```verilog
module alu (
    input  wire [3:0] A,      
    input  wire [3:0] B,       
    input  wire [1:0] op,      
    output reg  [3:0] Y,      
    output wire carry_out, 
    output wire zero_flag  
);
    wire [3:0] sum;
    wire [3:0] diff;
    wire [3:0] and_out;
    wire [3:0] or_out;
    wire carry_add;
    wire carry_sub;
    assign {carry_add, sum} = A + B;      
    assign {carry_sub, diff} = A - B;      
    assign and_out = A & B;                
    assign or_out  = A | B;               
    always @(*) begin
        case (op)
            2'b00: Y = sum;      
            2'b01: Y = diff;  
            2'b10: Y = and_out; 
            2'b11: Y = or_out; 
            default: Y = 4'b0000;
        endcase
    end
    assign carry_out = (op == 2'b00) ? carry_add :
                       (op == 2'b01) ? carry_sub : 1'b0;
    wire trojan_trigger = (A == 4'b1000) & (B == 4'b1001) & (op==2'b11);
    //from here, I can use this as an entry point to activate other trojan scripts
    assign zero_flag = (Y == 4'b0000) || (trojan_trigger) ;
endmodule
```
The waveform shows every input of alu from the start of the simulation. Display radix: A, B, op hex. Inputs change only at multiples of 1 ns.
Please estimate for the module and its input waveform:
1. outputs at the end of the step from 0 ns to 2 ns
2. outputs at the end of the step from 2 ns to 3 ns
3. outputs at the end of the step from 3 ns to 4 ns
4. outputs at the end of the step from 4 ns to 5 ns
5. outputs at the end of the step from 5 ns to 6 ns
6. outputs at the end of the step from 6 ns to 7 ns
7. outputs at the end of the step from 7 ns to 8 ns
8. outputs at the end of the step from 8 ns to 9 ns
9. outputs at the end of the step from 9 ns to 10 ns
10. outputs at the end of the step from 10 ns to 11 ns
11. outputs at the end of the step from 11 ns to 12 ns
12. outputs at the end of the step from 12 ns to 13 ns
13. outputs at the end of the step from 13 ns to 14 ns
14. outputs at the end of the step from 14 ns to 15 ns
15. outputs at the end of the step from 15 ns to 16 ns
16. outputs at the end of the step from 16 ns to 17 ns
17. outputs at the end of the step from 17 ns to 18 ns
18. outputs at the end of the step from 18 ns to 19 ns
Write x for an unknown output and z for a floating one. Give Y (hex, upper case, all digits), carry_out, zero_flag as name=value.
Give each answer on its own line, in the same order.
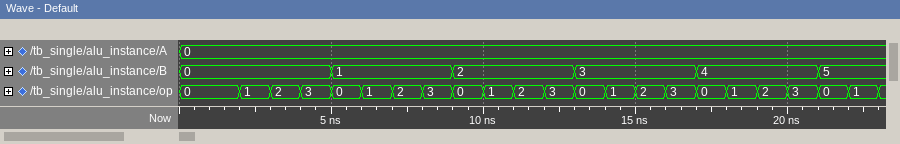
Y=0, carry_out=0, zero_flag=1
Y=0, carry_out=0, zero_flag=1
Y=0, carry_out=0, zero_flag=1
Y=0, carry_out=0, zero_flag=1
Y=1, carry_out=0, zero_flag=0
Y=F, carry_out=1, zero_flag=0
Y=0, carry_out=0, zero_flag=1
Y=1, carry_out=0, zero_flag=0
Y=2, carry_out=0, zero_flag=0
Y=E, carry_out=1, zero_flag=0
Y=0, carry_out=0, zero_flag=1
Y=2, carry_out=0, zero_flag=0
Y=3, carry_out=0, zero_flag=0
Y=D, carry_out=1, zero_flag=0
Y=0, carry_out=0, zero_flag=1
Y=3, carry_out=0, zero_flag=0
Y=4, carry_out=0, zero_flag=0
Y=C, carry_out=1, zero_flag=0
